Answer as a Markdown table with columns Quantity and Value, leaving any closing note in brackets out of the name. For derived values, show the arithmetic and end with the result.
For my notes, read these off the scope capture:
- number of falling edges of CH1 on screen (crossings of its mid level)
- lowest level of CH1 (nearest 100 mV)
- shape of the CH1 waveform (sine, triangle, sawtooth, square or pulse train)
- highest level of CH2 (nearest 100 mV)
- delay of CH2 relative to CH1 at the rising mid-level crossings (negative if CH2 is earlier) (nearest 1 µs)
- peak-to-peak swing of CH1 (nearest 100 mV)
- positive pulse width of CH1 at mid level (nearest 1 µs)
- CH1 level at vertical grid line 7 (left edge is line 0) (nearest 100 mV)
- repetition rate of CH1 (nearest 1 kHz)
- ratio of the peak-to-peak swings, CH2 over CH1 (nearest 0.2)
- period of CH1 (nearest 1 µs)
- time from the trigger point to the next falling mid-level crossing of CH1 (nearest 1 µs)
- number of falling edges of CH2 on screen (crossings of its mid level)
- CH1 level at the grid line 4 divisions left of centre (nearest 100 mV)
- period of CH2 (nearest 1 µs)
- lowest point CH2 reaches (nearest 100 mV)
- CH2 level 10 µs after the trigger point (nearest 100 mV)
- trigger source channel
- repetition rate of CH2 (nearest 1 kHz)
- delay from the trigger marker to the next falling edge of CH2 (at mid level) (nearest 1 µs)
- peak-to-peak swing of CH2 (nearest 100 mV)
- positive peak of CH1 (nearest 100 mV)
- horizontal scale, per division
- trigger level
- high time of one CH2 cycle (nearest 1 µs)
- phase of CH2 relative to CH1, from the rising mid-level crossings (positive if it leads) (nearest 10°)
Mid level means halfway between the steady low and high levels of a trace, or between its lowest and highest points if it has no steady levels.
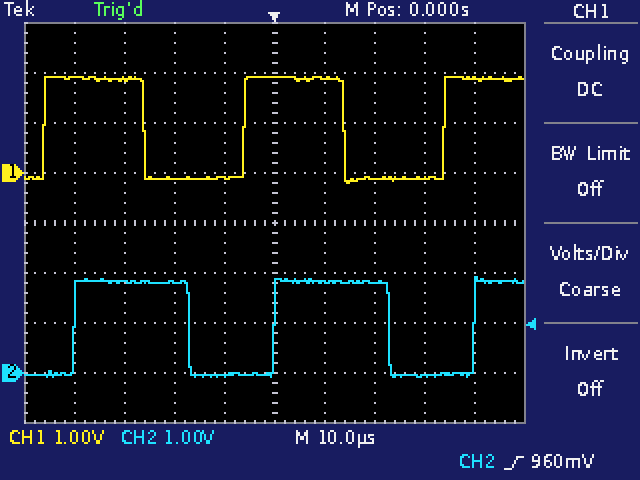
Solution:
| Quantity | Value |
|---|---|
| number of falling edges of CH1 on screen | 2 |
| lowest level of CH1 | -200 mV |
| shape of the CH1 waveform | square |
| highest level of CH2 | 1.9 V |
| delay of CH2 relative to CH1 at the rising mid-level crossings (negative if CH2 is earlier) | +6 µs |
| peak-to-peak swing of CH1 | 1.9 V − (-200 mV) = 2.1 V |
| positive pulse width of CH1 at mid level | 20 µs |
| CH1 level at vertical grid line 7 (left edge is line 0) | -100 mV |
| repetition rate of CH1 | 1 / 40 µs ≈ 25 kHz |
| ratio of the peak-to-peak swings, CH2 over CH1 | 2.0 V / 2.1 V ≈ 1.0 |
| period of CH1 | 40 µs |
| time from the trigger point to the next falling mid-level crossing of CH1 | 14 µs |
| number of falling edges of CH2 on screen | 2 |
| CH1 level at the grid line 4 divisions left of centre | 1.9 V |
| period of CH2 | 40 µs |
| lowest point CH2 reaches | -100 mV |
| CH2 level 10 µs after the trigger point | 1.8 V |
| trigger source channel | CH2 |
| repetition rate of CH2 | 1 / 40 µs ≈ 25 kHz |
| delay from the trigger marker to the next falling edge of CH2 (at mid level) | 23 µs |
| peak-to-peak swing of CH2 | 1.9 V − (-100 mV) = 2.0 V |
| positive peak of CH1 | 1.9 V |
| horizontal scale, per division | 10 µs |
| trigger level | 960 mV |
| high time of one CH2 cycle | 23 µs |
| phase of CH2 relative to CH1, from the rising mid-level crossings (positive if it leads) | −360° × (+6 µs) / 40 µs ≈ -54.0°, so -50° to the nearest 10° |
